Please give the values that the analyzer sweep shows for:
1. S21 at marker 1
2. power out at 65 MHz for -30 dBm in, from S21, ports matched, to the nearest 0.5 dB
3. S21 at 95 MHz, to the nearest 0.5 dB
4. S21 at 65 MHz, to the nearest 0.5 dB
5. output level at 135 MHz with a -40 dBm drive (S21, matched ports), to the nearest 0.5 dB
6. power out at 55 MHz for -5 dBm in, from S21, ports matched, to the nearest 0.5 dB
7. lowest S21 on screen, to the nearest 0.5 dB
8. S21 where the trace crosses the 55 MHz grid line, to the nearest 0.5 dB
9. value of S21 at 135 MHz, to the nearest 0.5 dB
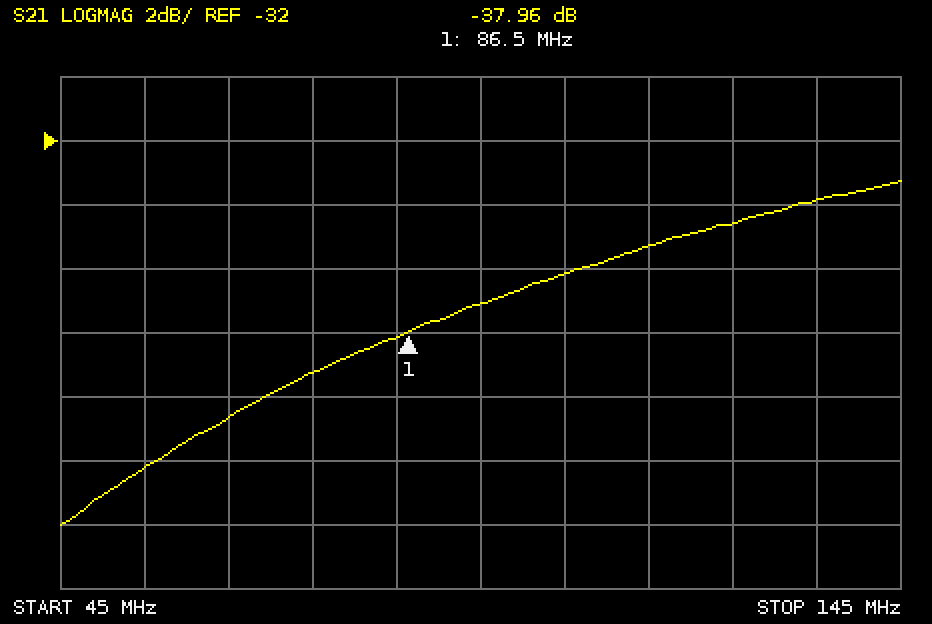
-37.96 dB
-70.5 dBm
-37.0 dB
-40.5 dB
-74.0 dBm
-47.0 dBm
-44.0 dB
-42.0 dB
-34.0 dB
